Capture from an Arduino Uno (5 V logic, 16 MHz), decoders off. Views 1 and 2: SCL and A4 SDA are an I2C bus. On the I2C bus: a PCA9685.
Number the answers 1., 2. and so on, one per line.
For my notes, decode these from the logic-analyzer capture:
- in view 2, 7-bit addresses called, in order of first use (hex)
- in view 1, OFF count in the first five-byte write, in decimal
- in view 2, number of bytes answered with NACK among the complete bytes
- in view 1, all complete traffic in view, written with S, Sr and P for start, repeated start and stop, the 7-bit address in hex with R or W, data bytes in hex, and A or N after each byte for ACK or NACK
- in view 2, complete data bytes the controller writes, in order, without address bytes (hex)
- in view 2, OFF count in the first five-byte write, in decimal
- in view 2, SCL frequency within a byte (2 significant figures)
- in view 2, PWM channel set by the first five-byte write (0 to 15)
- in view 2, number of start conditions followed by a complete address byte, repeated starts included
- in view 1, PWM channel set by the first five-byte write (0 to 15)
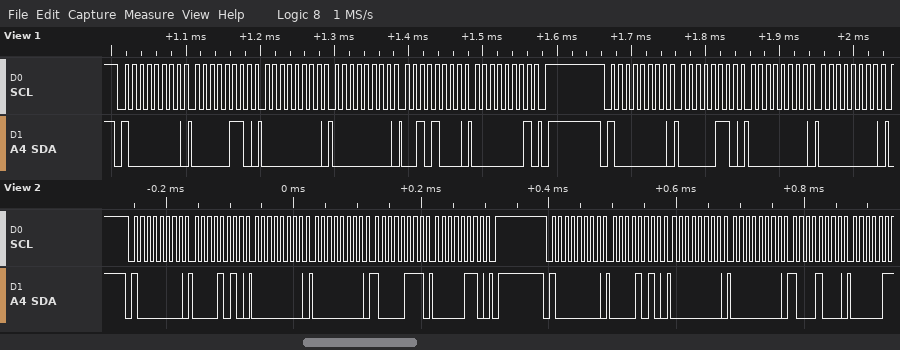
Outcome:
1. 0x40
2. 296
3. 0
4. S 40W A 06 A 00 A 00 A 28 A 01 A P S 40W A 06 A 00 A 00 A
5. 0A 00 00 87 06 0A 00 00 88
6. 1671
7. 100 kHz
8. 1
9. 2
10. 0
